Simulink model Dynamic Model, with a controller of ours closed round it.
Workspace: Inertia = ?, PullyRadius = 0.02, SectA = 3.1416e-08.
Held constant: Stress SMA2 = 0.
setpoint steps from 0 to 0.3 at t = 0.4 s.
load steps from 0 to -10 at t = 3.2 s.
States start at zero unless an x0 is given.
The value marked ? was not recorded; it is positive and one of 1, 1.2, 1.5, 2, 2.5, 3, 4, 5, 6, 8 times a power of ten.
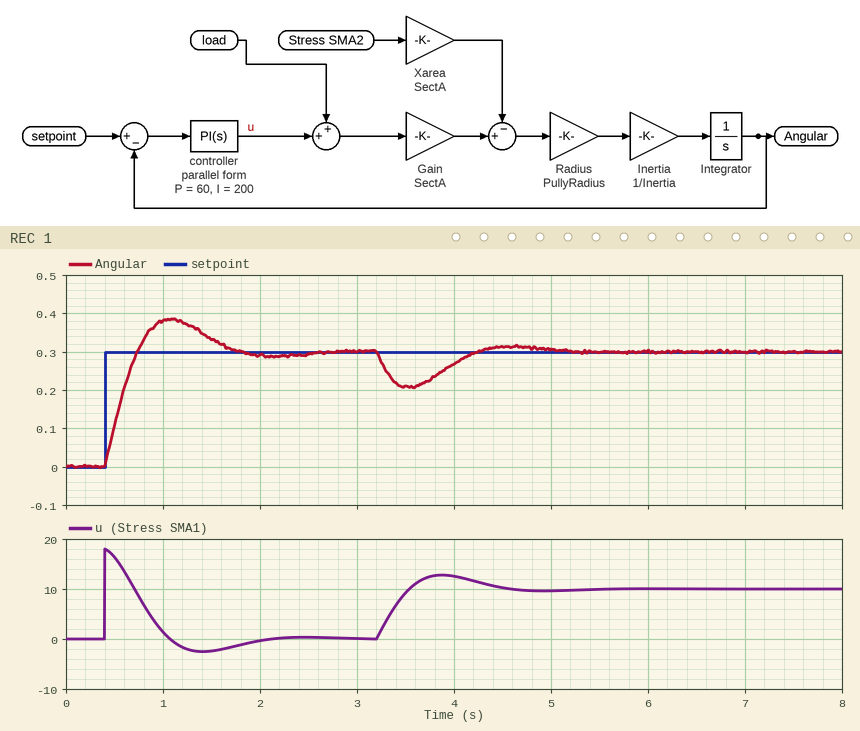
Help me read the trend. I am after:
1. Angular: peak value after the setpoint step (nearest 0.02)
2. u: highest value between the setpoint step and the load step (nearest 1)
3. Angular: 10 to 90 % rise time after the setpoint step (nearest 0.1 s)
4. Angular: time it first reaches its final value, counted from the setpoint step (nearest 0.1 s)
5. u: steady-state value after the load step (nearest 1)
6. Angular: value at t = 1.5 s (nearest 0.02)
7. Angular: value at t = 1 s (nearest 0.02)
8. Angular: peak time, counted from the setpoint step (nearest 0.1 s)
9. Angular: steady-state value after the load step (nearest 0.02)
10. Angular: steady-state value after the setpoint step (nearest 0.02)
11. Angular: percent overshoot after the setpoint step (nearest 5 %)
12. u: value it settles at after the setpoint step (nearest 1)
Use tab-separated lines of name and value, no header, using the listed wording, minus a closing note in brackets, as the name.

Angular: peak value after the setpoint step	0.38
u: highest value between the setpoint step and the load step	18
Angular: 10 to 90 % rise time after the setpoint step	0.3 s
Angular: time it first reaches its final value, counted from the setpoint step	0.3 s
u: steady-state value after the load step	10
Angular: value at t = 1.5 s	0.34
Angular: value at t = 1 s	0.38
Angular: peak time, counted from the setpoint step	0.7 s
Angular: steady-state value after the load step	0.30
Angular: steady-state value after the setpoint step	0.30
Angular: percent overshoot after the setpoint step	30 %
u: value it settles at after the setpoint step	0
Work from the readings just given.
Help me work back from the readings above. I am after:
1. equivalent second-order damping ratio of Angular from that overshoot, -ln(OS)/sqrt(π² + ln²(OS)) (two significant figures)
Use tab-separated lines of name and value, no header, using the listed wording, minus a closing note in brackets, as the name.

equivalent second-order damping ratio of Angular from that overshoot, -ln(OS)/sqrt(π² + ln²(OS))	0.36
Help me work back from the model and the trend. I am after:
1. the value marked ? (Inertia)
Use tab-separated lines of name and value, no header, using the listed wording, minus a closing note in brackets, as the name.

the value marked ?	1e-08
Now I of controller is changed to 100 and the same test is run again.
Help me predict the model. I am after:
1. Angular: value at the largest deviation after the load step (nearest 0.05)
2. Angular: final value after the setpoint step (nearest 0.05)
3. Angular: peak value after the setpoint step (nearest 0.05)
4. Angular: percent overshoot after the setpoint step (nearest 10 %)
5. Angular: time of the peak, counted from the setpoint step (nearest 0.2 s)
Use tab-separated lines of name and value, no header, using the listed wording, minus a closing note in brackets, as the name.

Angular: value at the largest deviation after the load step	0.20
Angular: final value after the setpoint step	0.30
Angular: peak value after the setpoint step	0.35
Angular: percent overshoot after the setpoint step	20 %
Angular: time of the peak, counted from the setpoint step	0.8 s
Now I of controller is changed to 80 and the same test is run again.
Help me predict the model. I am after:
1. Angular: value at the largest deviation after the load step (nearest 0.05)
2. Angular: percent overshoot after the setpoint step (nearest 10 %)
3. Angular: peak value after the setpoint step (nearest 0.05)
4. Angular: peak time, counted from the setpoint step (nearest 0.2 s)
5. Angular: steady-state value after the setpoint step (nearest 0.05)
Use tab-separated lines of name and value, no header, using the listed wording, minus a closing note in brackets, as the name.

Angular: value at the largest deviation after the load step	0.20
Angular: percent overshoot after the setpoint step	20 %
Angular: peak value after the setpoint step	0.35
Angular: peak time, counted from the setpoint step	1.0 s
Angular: steady-state value after the setpoint step	0.30
